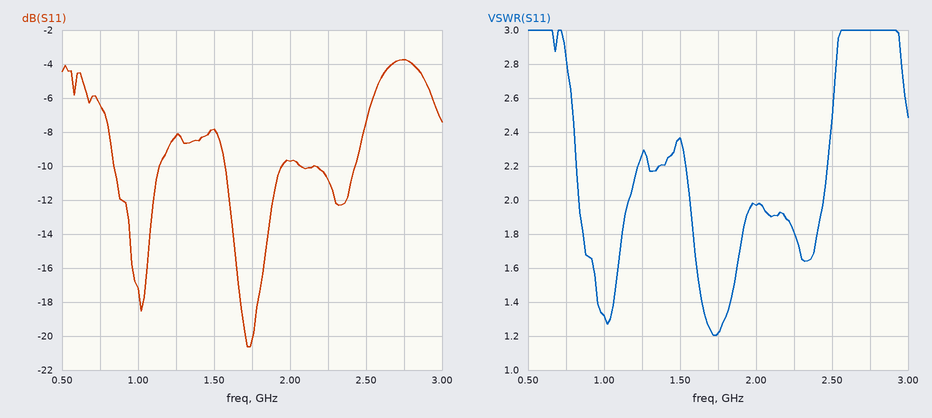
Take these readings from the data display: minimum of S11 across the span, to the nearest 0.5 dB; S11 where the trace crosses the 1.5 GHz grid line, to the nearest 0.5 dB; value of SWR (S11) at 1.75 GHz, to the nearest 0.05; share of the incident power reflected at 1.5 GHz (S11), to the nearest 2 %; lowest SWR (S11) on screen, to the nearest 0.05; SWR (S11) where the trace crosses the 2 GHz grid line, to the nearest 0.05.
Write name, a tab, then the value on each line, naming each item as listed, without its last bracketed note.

minimum of S11 across the span, to the nearest 0.5 dB	-20.5 dB
S11 where the trace crosses the 1.5 GHz grid line, to the nearest 0.5 dB	-8.0 dB
value of SWR (S11) at 1.75 GHz, to the nearest 0.05	1.20
share of the incident power reflected at 1.5 GHz (S11), to the nearest 2 %	16 %
lowest SWR (S11) on screen, to the nearest 0.05	1.20
SWR (S11) where the trace crosses the 2 GHz grid line, to the nearest 0.05	1.95
